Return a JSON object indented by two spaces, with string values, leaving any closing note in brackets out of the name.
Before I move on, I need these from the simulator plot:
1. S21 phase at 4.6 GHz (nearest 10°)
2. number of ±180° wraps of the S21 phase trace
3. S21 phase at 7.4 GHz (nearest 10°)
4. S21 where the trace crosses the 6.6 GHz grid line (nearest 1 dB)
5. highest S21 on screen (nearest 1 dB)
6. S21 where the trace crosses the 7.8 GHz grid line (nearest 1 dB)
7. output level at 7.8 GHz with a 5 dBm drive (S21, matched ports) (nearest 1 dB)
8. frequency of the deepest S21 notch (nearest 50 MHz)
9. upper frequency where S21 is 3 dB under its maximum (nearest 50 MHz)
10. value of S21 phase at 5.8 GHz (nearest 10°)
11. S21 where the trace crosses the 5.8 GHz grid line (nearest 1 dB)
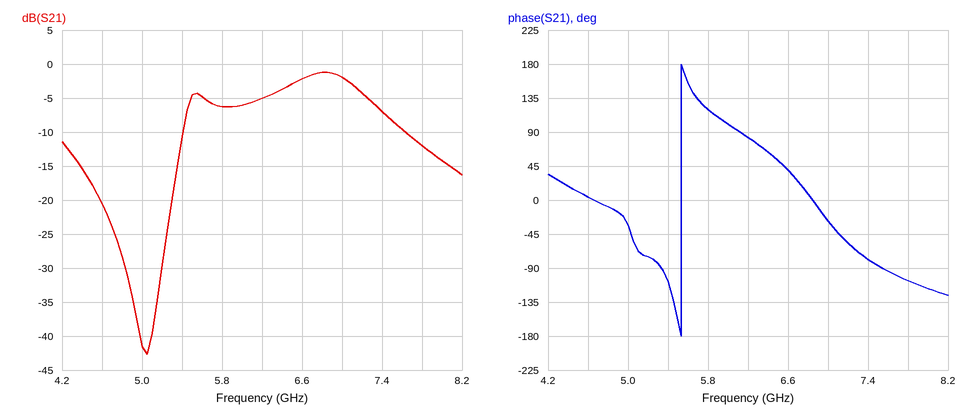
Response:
{
  "S21 phase at 4.6 GHz": "0°",
  "number of ±180° wraps of the S21 phase trace": "1",
  "S21 phase at 7.4 GHz": "-80°",
  "S21 where the trace crosses the 6.6 GHz grid line": "-2 dB",
  "highest S21 on screen": "-1 dB",
  "S21 where the trace crosses the 7.8 GHz grid line": "-12 dB",
  "output level at 7.8 GHz with a 5 dBm drive (S21, matched ports)": "-7 dBm",
  "frequency of the deepest S21 notch": "5.05 GHz",
  "upper frequency where S21 is 3 dB under its maximum": "7.20 GHz",
  "value of S21 phase at 5.8 GHz": "120°",
  "S21 where the trace crosses the 5.8 GHz grid line": "-6 dB"
}
